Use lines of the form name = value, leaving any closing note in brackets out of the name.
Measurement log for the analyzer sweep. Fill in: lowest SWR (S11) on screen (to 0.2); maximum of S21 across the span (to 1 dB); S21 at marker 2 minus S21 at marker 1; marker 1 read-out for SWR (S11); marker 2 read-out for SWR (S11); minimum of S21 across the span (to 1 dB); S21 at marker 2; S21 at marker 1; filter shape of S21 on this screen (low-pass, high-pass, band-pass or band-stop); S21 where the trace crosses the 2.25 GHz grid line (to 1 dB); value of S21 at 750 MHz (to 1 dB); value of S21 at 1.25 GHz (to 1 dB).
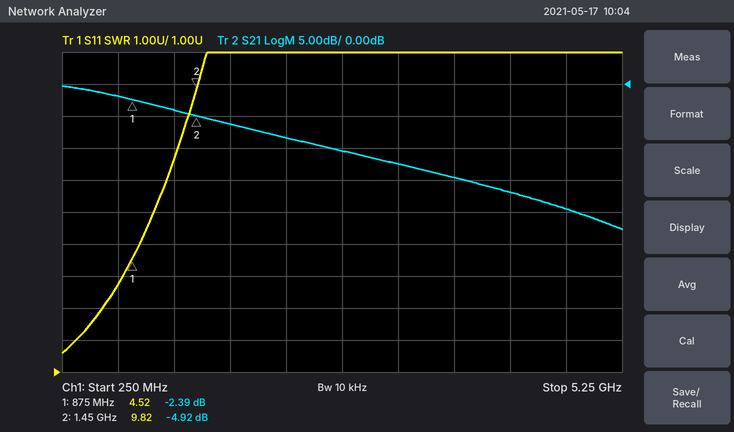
lowest SWR (S11) on screen = 1.6
maximum of S21 across the span = 0 dB
S21 at marker 2 minus S21 at marker 1 = -2.53 dB
marker 1 read-out for SWR = 4.52
marker 2 read-out for SWR = 9.82
minimum of S21 across the span = -23 dB
S21 at marker 2 = -4.92 dB
S21 at marker 1 = -2.39 dB
filter shape of S21 on this screen = low-pass
S21 where the trace crosses the 2.25 GHz grid line = -8 dB
value of S21 at 750 MHz = -2 dB
value of S21 at 1.25 GHz = -4 dB
